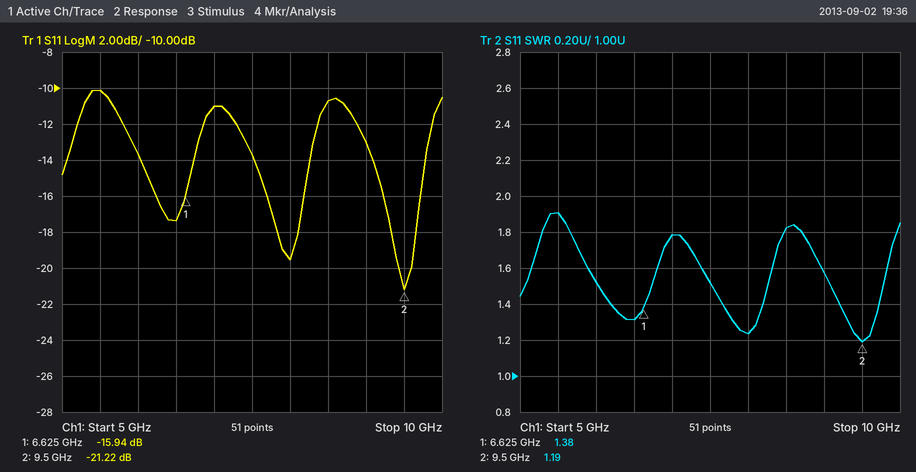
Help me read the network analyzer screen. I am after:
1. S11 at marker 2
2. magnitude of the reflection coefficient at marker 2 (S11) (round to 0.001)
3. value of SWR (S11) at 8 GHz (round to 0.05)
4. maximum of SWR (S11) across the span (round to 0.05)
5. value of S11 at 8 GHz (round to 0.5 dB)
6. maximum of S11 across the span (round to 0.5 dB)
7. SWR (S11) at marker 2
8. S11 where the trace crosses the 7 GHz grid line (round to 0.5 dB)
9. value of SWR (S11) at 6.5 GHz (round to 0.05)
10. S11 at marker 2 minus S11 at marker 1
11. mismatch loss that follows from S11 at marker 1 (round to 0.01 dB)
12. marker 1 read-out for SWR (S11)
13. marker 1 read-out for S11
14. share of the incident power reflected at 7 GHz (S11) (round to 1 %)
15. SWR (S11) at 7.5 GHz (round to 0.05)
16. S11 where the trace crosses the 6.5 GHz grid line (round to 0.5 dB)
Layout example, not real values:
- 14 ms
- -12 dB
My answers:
- -21.22 dB
- 0.087
- 1.25
- 1.90
- -19.5 dB
- -10.0 dB
- 1.19
- -11.0 dB
- 1.30
- -5.28 dB
- 0.11 dB
- 1.38
- -15.94 dB
- 8 %
- 1.50
- -17.5 dB
